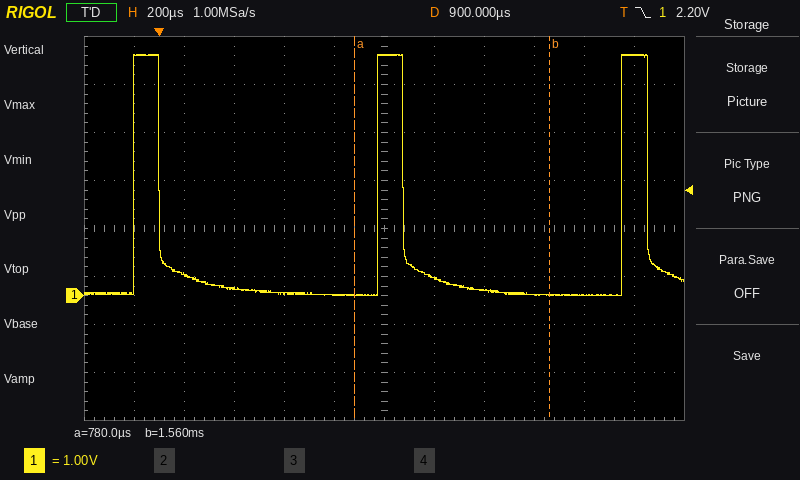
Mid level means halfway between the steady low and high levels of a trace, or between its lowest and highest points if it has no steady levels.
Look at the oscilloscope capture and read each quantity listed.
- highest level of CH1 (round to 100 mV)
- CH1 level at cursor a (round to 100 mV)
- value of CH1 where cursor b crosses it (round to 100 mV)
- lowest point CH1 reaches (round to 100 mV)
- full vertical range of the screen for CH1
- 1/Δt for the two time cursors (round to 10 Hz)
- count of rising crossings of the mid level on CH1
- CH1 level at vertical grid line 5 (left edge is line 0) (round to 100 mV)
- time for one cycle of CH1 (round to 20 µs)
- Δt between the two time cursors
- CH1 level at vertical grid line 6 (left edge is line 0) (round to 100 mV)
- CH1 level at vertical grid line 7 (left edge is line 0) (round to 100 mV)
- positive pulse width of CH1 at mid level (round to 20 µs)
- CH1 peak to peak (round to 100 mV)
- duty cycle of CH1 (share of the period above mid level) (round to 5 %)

5.0 V
0.0 V
0.0 V
0.0 V
8 V
1.28 kHz
3
0.0 V
980 µs
780 µs
5.0 V
400 mV
100 µs
5.0 V
10 %
